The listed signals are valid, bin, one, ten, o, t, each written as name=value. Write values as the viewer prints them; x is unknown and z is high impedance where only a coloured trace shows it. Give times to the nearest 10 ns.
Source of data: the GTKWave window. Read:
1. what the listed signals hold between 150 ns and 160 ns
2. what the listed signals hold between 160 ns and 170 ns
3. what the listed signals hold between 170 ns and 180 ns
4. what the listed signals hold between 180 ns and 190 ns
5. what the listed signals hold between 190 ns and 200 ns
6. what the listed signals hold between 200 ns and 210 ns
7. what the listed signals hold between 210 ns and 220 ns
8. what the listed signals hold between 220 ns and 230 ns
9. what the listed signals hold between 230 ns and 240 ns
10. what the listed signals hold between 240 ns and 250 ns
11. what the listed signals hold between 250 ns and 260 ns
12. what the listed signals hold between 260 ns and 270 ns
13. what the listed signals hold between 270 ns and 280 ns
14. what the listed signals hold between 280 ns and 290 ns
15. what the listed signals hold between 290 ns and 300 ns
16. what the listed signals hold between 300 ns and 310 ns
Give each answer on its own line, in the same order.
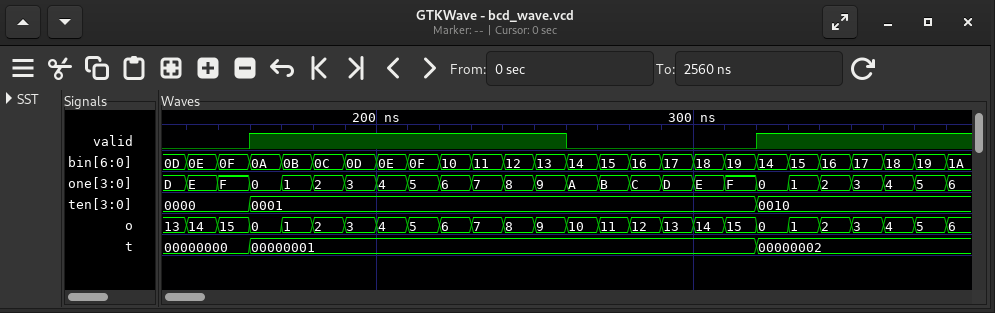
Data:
valid=0, bin=0F, one=F, ten=0000, o=15, t=00000000
valid=1, bin=0A, one=0, ten=0001, o=0, t=00000001
valid=1, bin=0B, one=1, ten=0001, o=1, t=00000001
valid=1, bin=0C, one=2, ten=0001, o=2, t=00000001
valid=1, bin=0D, one=3, ten=0001, o=3, t=00000001
valid=1, bin=0E, one=4, ten=0001, o=4, t=00000001
valid=1, bin=0F, one=5, ten=0001, o=5, t=00000001
valid=1, bin=10, one=6, ten=0001, o=6, t=00000001
valid=1, bin=11, one=7, ten=0001, o=7, t=00000001
valid=1, bin=12, one=8, ten=0001, o=8, t=00000001
valid=1, bin=13, one=9, ten=0001, o=9, t=00000001
valid=0, bin=14, one=A, ten=0001, o=10, t=00000001
valid=0, bin=15, one=B, ten=0001, o=11, t=00000001
valid=0, bin=16, one=C, ten=0001, o=12, t=00000001
valid=0, bin=17, one=D, ten=0001, o=13, t=00000001
valid=0, bin=18, one=E, ten=0001, o=14, t=00000001
